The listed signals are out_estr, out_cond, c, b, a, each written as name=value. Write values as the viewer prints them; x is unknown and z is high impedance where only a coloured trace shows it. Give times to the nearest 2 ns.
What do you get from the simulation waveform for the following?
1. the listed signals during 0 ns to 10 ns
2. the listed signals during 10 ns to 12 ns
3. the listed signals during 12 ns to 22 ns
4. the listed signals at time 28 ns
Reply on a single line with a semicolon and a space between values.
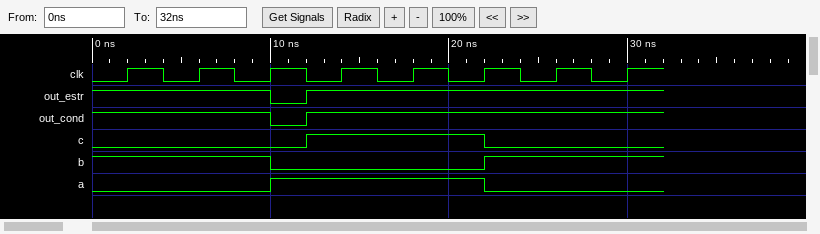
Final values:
out_estr=1, out_cond=1, c=0, b=1, a=0; out_estr=0, out_cond=0, c=0, b=0, a=1; out_estr=1, out_cond=1, c=1, b=0, a=1; out_estr=1, out_cond=1, c=0, b=1, a=0
